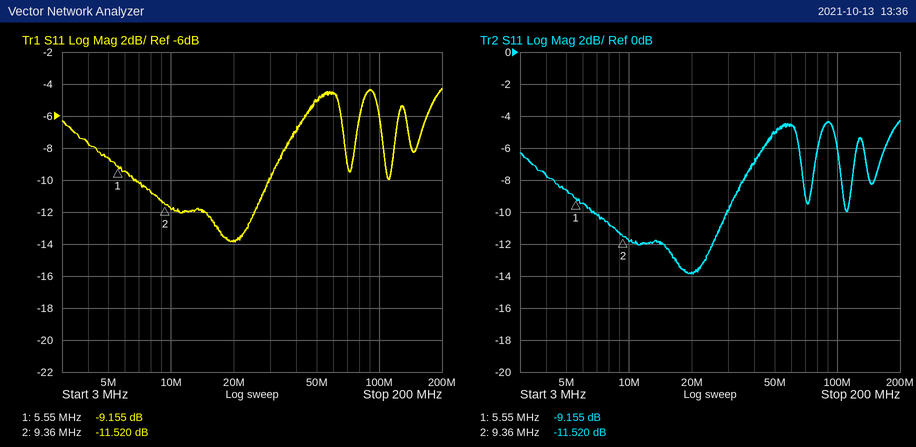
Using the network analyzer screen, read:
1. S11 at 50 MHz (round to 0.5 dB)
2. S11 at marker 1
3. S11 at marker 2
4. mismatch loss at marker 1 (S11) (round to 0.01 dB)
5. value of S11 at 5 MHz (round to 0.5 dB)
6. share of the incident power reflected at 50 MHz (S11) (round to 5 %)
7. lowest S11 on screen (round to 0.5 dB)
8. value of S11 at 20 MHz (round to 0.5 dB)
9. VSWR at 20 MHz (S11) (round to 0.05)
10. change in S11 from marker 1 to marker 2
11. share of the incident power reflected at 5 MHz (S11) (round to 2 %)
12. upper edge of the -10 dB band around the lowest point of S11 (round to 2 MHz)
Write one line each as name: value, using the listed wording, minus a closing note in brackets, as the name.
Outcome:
S11 at 50 MHz: -5.0 dB
S11 at marker 1: -9.155 dB
S11 at marker 2: -11.520 dB
mismatch loss at marker 1 (S11): 0.56 dB
value of S11 at 5 MHz: -8.5 dB
share of the incident power reflected at 50 MHz (S11): 30 %
lowest S11 on screen: -14.0 dB
value of S11 at 20 MHz: -14.0 dB
VSWR at 20 MHz (S11): 1.50
change in S11 from marker 1 to marker 2: -2.365 dB
share of the incident power reflected at 5 MHz (S11): 14 %
upper edge of the -10 dB band around the lowest point of S11: 30 MHz
